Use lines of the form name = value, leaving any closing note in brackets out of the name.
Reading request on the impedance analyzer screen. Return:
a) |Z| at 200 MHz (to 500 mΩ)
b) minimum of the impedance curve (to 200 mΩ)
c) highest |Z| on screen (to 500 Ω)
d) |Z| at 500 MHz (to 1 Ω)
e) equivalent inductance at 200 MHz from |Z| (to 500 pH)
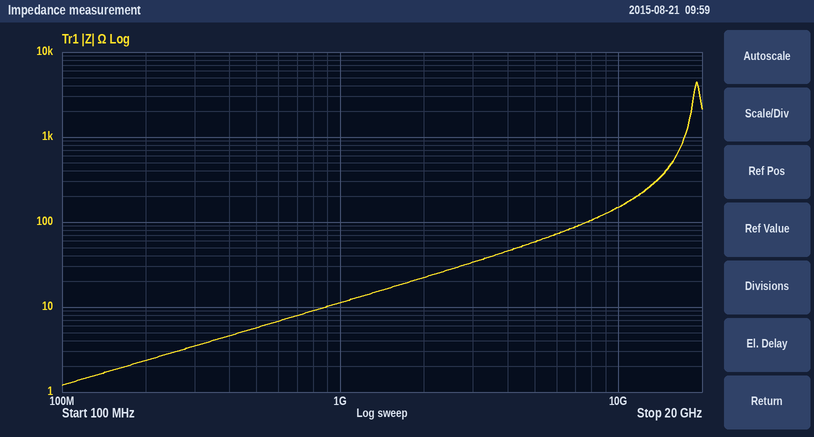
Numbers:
|Z| at 200 MHz = 2.5 Ω
minimum of the impedance curve = 1.2 Ω
highest |Z| on screen = 4.5 kΩ
|Z| at 500 MHz = 6 Ω
equivalent inductance at 200 MHz from |Z| = 2.0 nH
